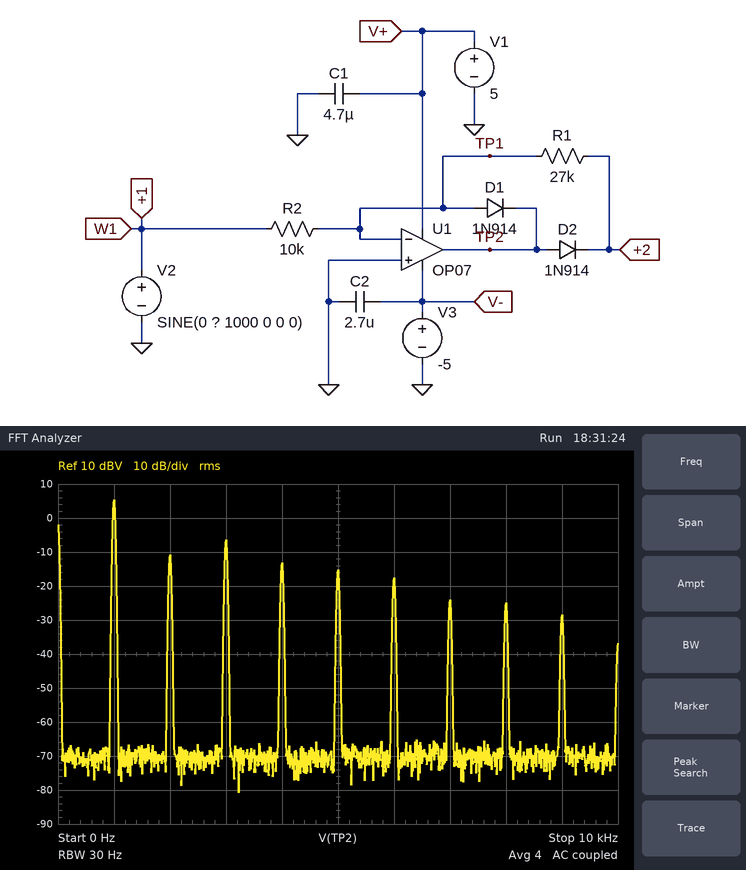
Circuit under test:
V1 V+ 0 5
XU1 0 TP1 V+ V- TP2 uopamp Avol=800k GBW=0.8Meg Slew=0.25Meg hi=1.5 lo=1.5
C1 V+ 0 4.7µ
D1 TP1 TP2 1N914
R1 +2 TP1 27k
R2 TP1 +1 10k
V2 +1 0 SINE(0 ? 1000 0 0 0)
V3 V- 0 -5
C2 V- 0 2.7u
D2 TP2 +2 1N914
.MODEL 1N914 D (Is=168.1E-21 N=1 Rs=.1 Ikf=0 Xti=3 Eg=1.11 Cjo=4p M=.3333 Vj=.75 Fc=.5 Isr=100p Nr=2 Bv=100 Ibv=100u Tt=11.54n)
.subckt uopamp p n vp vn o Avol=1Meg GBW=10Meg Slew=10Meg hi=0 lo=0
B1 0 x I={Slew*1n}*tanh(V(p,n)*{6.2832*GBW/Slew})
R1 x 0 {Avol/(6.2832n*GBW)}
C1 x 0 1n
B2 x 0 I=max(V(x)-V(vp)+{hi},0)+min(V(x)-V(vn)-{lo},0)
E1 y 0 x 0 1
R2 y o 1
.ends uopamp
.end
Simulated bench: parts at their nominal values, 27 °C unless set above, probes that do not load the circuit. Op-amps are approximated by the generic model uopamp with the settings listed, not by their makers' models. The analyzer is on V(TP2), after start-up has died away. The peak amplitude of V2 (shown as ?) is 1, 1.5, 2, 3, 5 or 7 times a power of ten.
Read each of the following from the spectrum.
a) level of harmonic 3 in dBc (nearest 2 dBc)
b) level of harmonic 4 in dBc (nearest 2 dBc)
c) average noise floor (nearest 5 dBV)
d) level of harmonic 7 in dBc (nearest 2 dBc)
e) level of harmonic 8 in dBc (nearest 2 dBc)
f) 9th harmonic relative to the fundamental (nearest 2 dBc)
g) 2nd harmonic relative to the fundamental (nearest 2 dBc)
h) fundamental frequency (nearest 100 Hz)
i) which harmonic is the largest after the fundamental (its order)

-12 dBc
-18 dBc
-70 dBV
-30 dBc
-30 dBc
-34 dBc
-16 dBc
1.0 kHz
3
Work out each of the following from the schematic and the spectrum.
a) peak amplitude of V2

2 V
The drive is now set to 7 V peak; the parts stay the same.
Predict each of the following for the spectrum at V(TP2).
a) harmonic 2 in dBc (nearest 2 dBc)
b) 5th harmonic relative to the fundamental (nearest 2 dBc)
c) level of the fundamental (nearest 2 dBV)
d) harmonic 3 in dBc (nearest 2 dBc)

-28 dBc
-14 dBc
6 dBV
-10 dBc
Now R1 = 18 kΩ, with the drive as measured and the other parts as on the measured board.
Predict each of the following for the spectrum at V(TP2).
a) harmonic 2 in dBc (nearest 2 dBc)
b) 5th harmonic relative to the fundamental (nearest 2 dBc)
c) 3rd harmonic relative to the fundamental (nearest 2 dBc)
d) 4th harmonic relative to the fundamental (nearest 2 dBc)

-14 dBc
-26 dBc
-14 dBc
-20 dBc
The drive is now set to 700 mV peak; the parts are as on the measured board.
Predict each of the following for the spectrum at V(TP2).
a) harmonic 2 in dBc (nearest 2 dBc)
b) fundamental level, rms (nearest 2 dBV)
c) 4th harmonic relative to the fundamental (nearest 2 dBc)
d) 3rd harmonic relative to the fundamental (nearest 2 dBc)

-14 dBc
2 dBV
-28 dBc
-16 dBc
